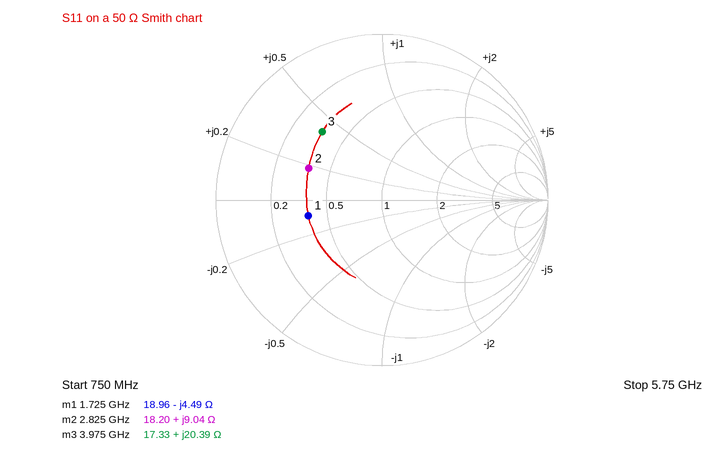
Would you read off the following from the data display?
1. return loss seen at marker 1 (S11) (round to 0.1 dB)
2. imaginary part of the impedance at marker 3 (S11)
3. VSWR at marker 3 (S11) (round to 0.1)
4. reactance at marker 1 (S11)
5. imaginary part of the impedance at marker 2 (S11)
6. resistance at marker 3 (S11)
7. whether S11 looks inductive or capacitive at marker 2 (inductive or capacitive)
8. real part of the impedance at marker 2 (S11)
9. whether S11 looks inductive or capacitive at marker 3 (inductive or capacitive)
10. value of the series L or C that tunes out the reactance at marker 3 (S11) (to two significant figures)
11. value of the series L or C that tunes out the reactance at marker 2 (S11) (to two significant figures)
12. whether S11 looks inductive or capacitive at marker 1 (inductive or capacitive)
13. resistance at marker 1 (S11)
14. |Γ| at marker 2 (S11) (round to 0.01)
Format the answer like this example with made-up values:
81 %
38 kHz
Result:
6.9 dB
+20.39 Ω
3.4
-4.49 Ω
+9.04 Ω
17.33 Ω
inductive
18.20 Ω
inductive
2.0 pF
6.2 pF
capacitive
18.96 Ω
0.48
